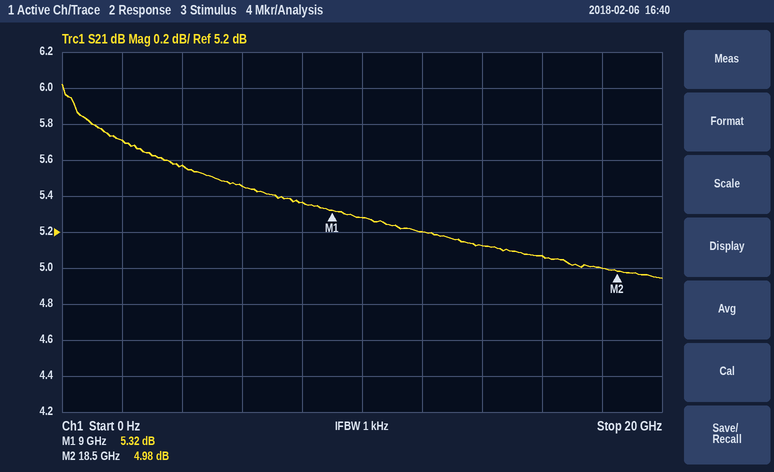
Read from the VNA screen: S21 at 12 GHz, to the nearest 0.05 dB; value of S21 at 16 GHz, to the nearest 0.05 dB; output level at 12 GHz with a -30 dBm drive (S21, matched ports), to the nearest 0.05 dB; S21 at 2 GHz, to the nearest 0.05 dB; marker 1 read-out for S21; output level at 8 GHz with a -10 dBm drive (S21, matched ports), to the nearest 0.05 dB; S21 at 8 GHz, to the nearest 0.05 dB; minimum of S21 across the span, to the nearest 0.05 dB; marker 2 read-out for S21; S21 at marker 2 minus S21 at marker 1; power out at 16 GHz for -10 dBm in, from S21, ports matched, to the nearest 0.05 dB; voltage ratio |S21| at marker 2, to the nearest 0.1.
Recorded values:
5.20 dB
5.05 dB
-24.80 dBm
5.70 dB
5.32 dB
-4.65 dBm
5.35 dB
4.95 dB
4.98 dB
-0.34 dB
-4.95 dBm
1.8
